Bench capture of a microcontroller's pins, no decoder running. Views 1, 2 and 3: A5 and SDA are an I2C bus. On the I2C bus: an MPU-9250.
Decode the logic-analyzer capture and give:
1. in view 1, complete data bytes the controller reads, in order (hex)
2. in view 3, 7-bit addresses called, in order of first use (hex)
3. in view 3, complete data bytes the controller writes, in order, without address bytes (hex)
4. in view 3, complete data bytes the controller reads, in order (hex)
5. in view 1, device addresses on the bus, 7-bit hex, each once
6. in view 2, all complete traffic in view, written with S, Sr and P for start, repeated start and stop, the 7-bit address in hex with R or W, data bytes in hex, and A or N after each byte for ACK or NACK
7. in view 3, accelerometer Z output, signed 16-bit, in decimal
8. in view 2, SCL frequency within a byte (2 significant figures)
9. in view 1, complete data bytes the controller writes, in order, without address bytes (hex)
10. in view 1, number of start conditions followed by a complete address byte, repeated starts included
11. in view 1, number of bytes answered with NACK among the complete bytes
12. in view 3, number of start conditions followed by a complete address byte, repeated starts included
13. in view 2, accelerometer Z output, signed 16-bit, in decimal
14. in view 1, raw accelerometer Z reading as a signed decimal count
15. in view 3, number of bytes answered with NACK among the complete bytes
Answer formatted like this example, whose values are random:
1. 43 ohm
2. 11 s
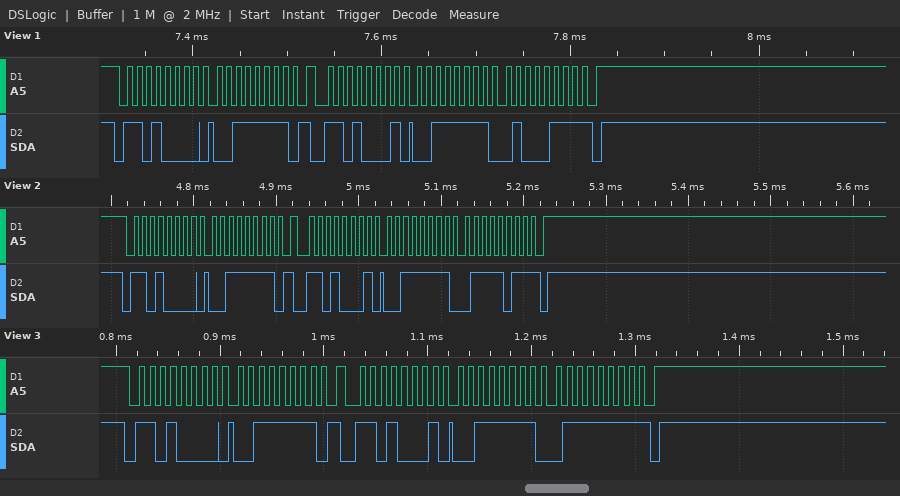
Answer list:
1. 3F 47
2. 0x68
3. 3F
4. 3F 7F
5. 0x68
6. S 68W A 3F A Sr 68R A 3F A 7B N P
7. 16255
8. 100 kHz
9. 3F
10. 2
11. 1
12. 2
13. 16251
14. 16199
15. 1
